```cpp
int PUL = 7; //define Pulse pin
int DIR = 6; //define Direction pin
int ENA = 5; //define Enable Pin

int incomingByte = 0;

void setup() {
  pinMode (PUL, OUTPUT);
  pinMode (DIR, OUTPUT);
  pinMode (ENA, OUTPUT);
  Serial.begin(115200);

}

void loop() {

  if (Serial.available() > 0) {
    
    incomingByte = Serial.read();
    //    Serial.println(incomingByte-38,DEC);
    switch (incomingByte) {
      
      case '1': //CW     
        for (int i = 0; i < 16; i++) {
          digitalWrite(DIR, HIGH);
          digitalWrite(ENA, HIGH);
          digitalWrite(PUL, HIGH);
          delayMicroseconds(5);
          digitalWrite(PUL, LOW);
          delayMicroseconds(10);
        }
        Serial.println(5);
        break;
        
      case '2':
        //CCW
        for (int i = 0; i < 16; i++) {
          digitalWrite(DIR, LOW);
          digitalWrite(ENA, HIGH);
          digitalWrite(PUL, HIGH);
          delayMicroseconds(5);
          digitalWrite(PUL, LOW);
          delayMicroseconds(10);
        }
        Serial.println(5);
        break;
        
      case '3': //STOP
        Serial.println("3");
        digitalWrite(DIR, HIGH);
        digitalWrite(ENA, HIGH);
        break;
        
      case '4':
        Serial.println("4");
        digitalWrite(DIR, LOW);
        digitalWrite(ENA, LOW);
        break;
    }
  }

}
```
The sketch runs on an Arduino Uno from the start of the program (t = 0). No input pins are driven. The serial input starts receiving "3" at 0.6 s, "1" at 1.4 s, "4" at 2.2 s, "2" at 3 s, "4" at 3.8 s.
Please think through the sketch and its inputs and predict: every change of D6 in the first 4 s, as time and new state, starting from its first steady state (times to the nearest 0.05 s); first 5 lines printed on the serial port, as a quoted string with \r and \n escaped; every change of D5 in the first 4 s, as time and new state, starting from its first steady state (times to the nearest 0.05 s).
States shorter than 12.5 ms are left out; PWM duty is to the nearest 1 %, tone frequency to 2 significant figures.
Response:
0 s low; 0.6 s high; 2.2 s low
"3\r\n5\r\n4\r\n5\r\n4\r\n"
0 s low; 0.6 s high; 2.2 s low; 3 s high; 3.8 s low
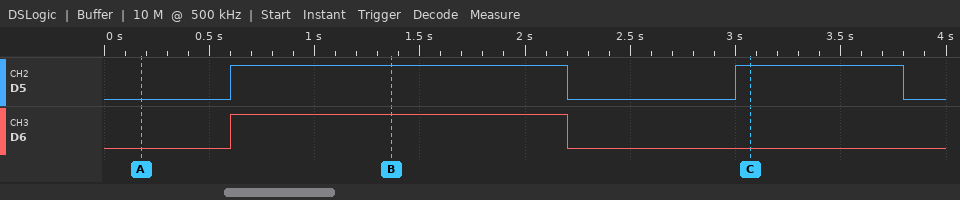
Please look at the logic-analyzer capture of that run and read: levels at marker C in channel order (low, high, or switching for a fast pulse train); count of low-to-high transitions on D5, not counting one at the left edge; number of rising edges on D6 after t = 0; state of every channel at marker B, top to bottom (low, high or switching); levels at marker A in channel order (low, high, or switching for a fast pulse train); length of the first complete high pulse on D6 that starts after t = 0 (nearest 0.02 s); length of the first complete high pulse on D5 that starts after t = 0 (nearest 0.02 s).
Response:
D5 high, D6 low
2
1
D5 high, D6 high
D5 low, D6 low
1.60 s
1.60 s
